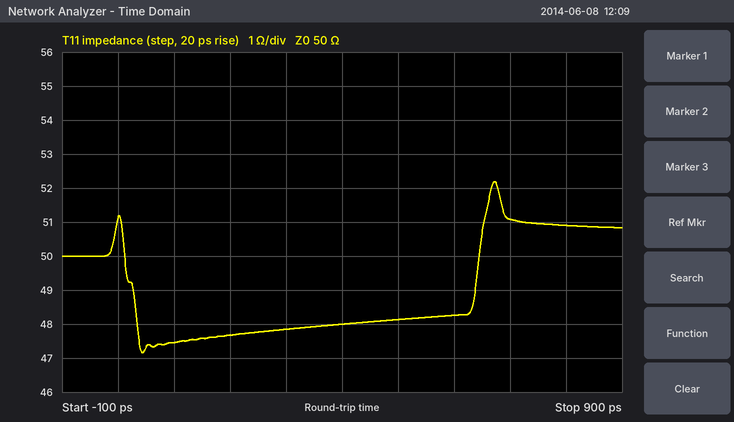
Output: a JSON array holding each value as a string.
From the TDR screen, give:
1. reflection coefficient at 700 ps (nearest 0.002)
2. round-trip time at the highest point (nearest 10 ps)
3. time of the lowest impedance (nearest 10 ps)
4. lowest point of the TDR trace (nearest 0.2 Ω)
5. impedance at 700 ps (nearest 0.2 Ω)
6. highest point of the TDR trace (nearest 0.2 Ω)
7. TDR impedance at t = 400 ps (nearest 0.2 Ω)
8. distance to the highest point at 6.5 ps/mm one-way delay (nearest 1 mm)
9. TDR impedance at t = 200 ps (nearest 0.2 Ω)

["+0.010", "670 ps", "40 ps", "47.2 Ω", "51.0 Ω", "52.2 Ω", "48.0 Ω", "52 mm", "47.6 Ω"]
